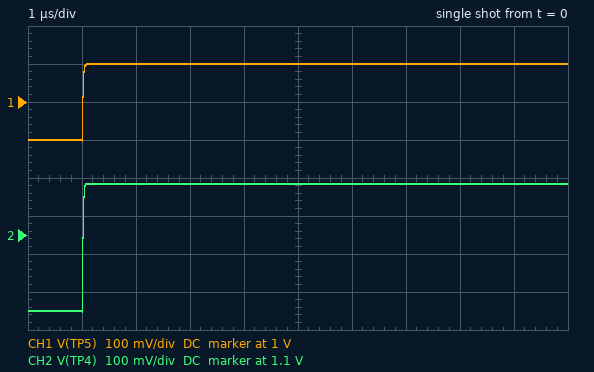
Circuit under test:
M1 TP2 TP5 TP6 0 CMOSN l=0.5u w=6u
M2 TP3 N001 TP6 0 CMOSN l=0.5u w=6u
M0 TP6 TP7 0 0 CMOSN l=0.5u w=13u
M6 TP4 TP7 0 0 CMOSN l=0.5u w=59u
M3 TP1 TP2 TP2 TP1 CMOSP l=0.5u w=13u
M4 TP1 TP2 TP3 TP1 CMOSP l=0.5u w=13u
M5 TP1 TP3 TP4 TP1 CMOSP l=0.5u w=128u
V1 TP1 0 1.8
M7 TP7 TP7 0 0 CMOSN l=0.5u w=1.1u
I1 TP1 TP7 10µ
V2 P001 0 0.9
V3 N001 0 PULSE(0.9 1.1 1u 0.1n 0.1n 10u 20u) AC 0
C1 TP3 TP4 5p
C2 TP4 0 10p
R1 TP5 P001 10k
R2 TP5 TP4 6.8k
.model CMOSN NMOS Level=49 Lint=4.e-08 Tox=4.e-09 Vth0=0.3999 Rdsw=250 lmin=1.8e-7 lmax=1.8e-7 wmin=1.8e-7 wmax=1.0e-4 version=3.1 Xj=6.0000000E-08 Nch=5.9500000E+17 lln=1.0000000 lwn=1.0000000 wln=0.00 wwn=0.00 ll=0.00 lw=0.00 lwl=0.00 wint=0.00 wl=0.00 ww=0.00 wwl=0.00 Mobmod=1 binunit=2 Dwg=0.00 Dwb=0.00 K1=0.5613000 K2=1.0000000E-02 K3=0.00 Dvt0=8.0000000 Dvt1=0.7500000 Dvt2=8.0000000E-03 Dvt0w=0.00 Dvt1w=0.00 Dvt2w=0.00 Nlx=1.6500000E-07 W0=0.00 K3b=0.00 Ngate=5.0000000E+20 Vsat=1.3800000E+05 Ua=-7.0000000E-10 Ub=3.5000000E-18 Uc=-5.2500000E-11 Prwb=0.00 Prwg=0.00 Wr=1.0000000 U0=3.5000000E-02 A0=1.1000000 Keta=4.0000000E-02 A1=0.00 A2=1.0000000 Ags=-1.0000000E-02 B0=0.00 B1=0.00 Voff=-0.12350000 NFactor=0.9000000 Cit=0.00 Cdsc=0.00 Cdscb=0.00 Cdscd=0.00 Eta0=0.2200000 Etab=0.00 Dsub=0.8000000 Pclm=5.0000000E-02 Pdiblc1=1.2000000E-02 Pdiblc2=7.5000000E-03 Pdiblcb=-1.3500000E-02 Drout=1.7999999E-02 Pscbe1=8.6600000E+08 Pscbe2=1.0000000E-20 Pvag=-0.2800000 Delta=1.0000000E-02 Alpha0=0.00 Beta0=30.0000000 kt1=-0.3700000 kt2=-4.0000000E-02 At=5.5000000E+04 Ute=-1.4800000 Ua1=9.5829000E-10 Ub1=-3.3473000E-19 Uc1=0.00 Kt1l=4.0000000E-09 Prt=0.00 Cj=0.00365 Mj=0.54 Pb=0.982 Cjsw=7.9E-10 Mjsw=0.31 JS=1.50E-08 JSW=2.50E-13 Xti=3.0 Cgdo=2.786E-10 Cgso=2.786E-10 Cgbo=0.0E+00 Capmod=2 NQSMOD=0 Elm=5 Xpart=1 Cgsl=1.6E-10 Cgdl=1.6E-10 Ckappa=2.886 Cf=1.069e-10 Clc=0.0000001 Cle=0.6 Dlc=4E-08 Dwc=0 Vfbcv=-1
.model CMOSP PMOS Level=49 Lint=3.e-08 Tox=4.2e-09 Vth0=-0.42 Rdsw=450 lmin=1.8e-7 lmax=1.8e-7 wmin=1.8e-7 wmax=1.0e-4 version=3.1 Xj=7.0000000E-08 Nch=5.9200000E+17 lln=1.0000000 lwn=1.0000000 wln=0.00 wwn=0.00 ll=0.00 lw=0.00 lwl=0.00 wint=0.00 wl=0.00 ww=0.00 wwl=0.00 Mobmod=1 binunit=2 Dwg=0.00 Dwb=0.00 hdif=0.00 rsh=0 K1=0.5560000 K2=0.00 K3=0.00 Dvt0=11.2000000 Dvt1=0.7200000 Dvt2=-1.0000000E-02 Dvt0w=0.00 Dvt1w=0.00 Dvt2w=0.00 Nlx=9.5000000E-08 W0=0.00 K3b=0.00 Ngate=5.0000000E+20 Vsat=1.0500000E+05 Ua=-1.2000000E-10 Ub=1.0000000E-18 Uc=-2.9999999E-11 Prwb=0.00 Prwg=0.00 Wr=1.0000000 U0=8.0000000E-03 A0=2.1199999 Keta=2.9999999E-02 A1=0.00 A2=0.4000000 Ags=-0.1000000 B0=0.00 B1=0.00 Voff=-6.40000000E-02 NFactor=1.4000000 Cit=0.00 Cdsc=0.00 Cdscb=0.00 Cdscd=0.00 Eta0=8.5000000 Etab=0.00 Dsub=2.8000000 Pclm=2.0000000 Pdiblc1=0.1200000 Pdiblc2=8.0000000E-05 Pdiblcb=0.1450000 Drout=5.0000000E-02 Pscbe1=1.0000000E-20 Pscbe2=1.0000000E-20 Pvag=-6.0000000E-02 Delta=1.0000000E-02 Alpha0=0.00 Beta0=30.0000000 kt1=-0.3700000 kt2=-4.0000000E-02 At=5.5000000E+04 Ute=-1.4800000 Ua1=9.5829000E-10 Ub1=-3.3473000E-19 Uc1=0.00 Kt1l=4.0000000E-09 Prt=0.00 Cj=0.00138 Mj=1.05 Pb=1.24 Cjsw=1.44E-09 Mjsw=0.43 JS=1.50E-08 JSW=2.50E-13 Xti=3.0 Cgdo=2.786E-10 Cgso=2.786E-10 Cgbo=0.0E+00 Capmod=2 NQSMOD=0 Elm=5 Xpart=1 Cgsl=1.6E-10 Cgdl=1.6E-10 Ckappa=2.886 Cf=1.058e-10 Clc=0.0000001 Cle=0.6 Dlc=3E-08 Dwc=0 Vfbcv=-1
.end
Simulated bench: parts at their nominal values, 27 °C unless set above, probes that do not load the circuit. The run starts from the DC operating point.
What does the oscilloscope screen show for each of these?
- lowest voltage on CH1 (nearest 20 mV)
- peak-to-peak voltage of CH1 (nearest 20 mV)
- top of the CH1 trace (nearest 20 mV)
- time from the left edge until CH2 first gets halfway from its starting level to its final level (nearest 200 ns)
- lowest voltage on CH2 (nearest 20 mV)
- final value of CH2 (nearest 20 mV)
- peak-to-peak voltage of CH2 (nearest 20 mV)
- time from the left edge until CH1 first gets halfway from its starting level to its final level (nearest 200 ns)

900 mV
200 mV
1.10 V
1.0 µs
900 mV
1.24 V
340 mV
1.0 µs
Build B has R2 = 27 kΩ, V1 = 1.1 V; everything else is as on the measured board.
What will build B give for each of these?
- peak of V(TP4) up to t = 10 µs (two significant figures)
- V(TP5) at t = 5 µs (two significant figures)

990 mV
920 mV
